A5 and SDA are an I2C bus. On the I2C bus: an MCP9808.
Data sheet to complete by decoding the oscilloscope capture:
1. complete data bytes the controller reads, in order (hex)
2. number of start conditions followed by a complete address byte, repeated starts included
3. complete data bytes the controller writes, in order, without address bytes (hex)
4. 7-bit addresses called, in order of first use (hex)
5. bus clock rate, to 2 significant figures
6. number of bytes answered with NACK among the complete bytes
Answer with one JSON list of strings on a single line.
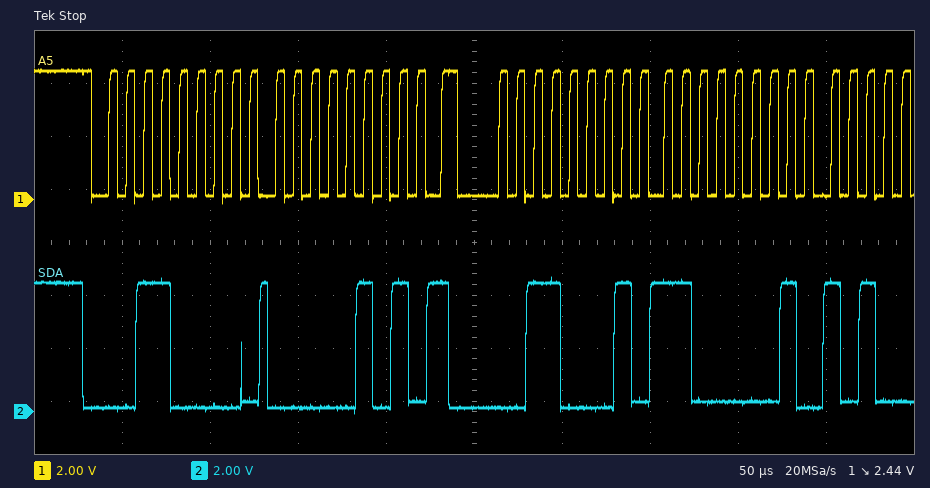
["C1", "2", "05", "0x18", "100 kHz", "0"]
